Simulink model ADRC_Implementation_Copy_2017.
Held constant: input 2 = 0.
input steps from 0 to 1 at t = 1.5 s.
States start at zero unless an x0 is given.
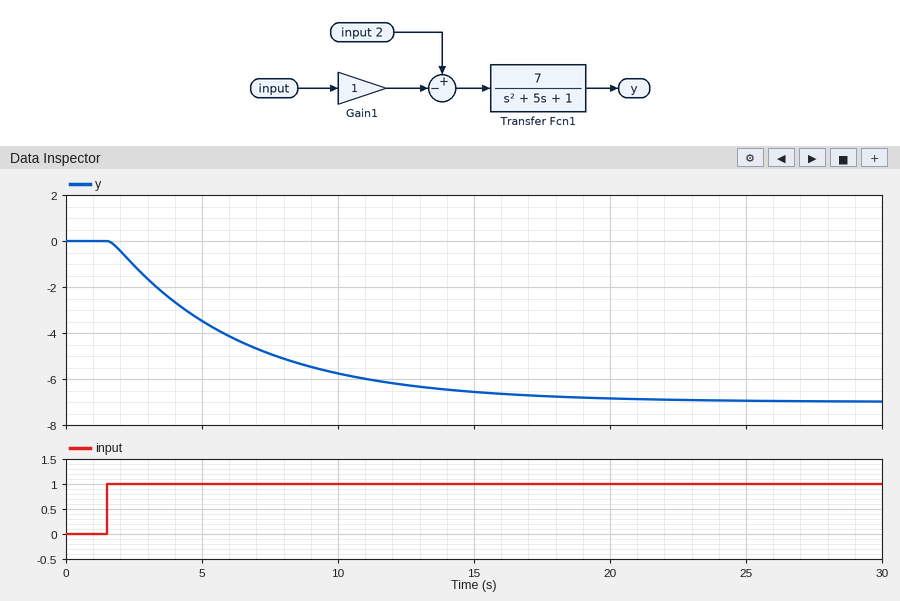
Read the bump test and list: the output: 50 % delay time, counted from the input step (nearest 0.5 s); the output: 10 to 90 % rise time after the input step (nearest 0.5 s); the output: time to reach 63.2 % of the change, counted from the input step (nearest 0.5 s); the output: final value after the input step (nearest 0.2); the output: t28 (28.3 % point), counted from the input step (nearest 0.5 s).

3.5 s
10.5 s
5.0 s
-7.0
2.0 s
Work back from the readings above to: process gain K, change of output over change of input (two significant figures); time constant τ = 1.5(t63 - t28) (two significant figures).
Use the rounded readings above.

-7.0
4.5 s
